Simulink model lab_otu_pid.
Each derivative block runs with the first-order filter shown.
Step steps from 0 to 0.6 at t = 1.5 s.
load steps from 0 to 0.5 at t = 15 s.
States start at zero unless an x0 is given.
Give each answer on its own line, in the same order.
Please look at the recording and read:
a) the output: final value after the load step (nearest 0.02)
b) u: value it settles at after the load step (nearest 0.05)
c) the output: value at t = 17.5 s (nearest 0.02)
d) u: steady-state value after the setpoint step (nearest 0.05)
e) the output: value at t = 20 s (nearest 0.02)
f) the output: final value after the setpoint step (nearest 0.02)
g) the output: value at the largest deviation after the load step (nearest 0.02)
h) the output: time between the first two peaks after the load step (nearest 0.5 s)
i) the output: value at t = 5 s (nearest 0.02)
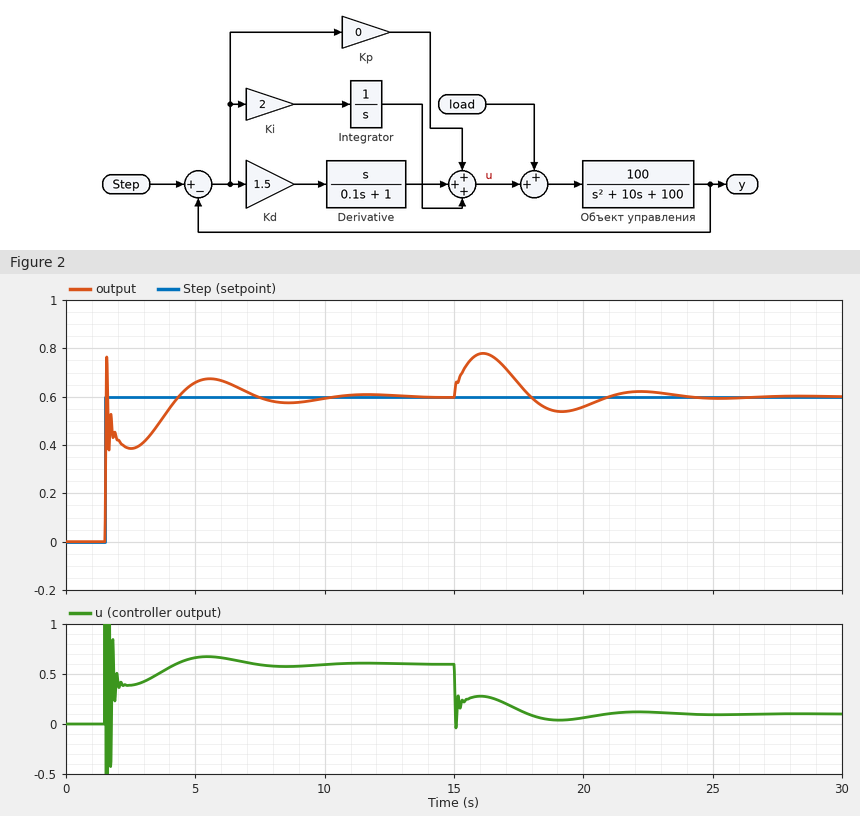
0.60
0.10
0.66
0.60
0.56
0.60
0.78
6.0 s
0.66
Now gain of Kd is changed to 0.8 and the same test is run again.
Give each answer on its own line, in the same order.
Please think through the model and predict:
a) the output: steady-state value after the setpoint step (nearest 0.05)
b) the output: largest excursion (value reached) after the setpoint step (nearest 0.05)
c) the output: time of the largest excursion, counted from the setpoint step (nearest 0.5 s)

0.60
0.65
3.0 s
